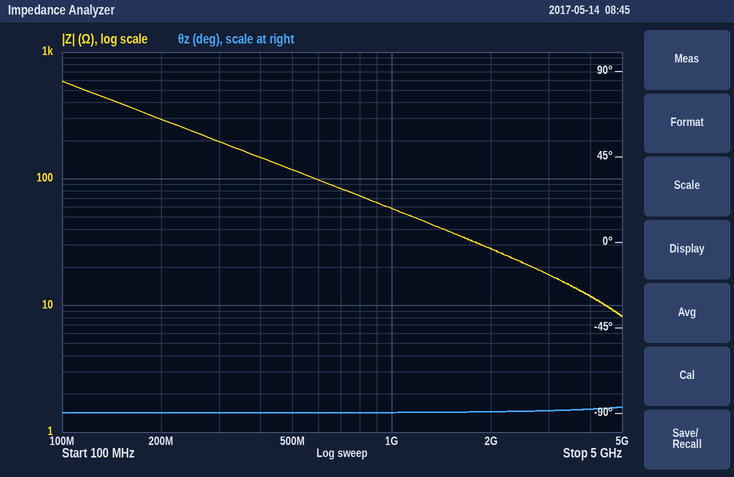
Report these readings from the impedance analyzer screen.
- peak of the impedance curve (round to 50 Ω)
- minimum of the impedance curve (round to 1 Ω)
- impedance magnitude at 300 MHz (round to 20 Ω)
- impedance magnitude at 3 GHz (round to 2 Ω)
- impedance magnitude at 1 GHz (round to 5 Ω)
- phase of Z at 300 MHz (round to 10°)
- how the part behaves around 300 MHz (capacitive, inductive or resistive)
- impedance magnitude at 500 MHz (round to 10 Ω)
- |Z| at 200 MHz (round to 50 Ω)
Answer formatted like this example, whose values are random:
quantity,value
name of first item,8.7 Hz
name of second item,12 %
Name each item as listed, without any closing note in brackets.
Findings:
quantity,value
peak of the impedance curve,600 Ω
minimum of the impedance curve,8 Ω
impedance magnitude at 300 MHz,200 Ω
impedance magnitude at 3 GHz,18 Ω
impedance magnitude at 1 GHz,60 Ω
phase of Z at 300 MHz,-90°
how the part behaves around 300 MHz,capacitive
impedance magnitude at 500 MHz,120 Ω
|Z| at 200 MHz,300 Ω
